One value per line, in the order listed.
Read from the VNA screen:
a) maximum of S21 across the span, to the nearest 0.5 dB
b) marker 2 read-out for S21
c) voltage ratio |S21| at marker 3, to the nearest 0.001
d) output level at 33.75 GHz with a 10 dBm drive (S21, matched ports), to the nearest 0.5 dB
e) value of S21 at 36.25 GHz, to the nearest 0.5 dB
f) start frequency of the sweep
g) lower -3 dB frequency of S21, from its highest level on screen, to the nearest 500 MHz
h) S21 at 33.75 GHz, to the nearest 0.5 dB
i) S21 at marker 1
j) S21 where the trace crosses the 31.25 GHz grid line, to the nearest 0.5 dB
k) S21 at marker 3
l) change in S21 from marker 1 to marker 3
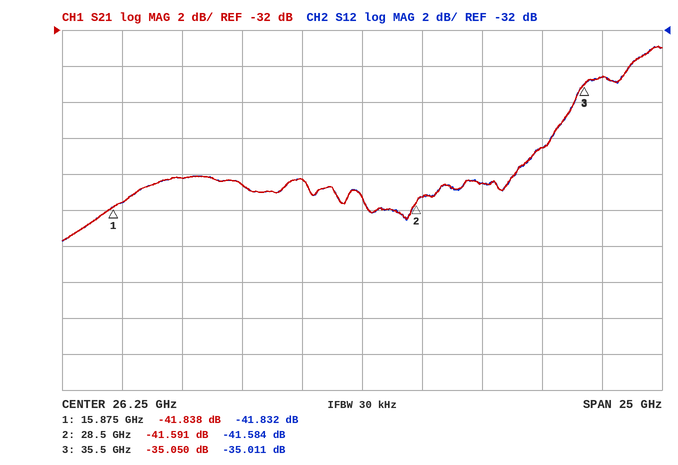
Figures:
-33.0 dB
-41.591 dB
0.018
-28.5 dBm
-34.5 dB
13.75 GHz
35.0 GHz
-38.5 dB
-41.838 dB
-40.5 dB
-35.050 dB
6.788 dB
